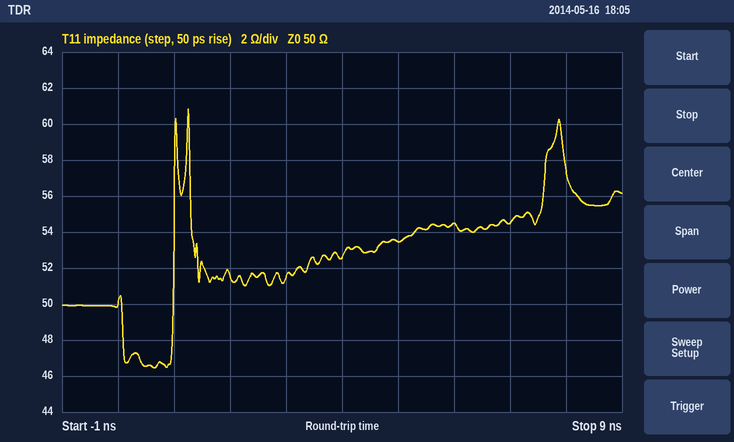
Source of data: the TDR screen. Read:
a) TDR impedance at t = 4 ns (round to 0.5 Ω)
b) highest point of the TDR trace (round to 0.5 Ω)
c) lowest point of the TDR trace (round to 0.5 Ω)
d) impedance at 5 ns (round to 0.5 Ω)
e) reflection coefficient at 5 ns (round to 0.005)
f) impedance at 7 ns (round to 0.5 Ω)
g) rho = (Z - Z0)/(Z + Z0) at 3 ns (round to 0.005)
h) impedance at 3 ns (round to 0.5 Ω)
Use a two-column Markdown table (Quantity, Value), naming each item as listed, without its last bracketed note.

| Quantity | Value |
|---|---|
| TDR impedance at t = 4 ns | 52.5 Ω |
| highest point of the TDR trace | 61.0 Ω |
| lowest point of the TDR trace | 46.5 Ω |
| impedance at 5 ns | 53.5 Ω |
| reflection coefficient at 5 ns | +0.035 |
| impedance at 7 ns | 54.5 Ω |
| rho = (Z - Z0)/(Z + Z0) at 3 ns | +0.015 |
| impedance at 3 ns | 51.5 Ω |
